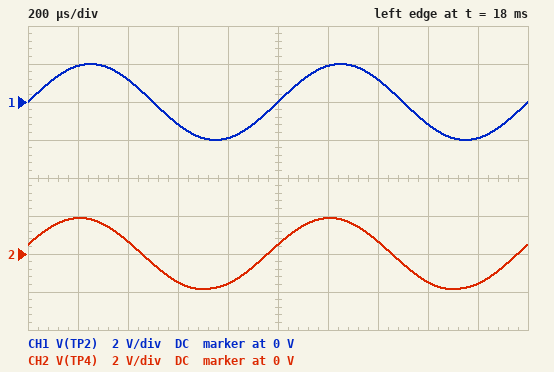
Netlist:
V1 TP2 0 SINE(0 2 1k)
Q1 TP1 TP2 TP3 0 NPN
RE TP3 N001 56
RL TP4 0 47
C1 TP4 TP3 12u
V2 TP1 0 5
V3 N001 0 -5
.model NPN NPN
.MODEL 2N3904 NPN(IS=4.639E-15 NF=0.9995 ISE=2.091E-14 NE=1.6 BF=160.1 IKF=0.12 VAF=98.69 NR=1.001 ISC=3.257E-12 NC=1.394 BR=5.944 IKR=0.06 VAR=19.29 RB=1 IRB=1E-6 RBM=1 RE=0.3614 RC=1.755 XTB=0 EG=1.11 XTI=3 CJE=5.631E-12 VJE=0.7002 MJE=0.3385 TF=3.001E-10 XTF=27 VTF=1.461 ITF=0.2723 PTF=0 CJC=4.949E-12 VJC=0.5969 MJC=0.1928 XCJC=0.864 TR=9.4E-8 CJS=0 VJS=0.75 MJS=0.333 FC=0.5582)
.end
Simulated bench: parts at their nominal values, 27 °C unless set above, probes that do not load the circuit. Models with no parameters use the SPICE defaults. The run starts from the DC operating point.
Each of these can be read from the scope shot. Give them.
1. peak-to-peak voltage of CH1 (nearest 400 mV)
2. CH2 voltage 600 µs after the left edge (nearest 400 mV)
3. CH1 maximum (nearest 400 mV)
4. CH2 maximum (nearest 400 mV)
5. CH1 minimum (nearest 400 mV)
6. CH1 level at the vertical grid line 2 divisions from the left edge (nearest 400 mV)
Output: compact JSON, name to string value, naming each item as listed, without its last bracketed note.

{"peak-to-peak voltage of CH1": "4.0 V", "CH2 voltage 600 µs after the left edge": "-1.6 V", "CH1 maximum": "2.0 V", "CH2 maximum": "2.0 V", "CH1 minimum": "-2.0 V", "CH1 level at the vertical grid line 2 divisions from the left edge": "1.2 V"}
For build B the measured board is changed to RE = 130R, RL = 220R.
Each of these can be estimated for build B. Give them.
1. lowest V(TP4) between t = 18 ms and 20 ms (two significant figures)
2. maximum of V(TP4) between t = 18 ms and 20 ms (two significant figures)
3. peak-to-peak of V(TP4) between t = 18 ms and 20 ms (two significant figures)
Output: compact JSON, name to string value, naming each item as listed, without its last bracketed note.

{"lowest V(TP4) between t = 18 ms and 20 ms": "-2.0 V", "maximum of V(TP4) between t = 18 ms and 20 ms": "2.0 V", "peak-to-peak of V(TP4) between t = 18 ms and 20 ms": "3.9 V"}
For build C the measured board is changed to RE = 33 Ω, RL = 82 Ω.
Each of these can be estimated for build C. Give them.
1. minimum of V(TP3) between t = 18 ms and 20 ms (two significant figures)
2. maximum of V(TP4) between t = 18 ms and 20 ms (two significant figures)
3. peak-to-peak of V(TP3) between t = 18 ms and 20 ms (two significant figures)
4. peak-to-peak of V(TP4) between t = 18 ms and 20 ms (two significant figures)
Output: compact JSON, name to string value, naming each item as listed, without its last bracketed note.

{"minimum of V(TP3) between t = 18 ms and 20 ms": "-2.9 V", "maximum of V(TP4) between t = 18 ms and 20 ms": "2.0 V", "peak-to-peak of V(TP3) between t = 18 ms and 20 ms": "4.0 V", "peak-to-peak of V(TP4) between t = 18 ms and 20 ms": "3.9 V"}
